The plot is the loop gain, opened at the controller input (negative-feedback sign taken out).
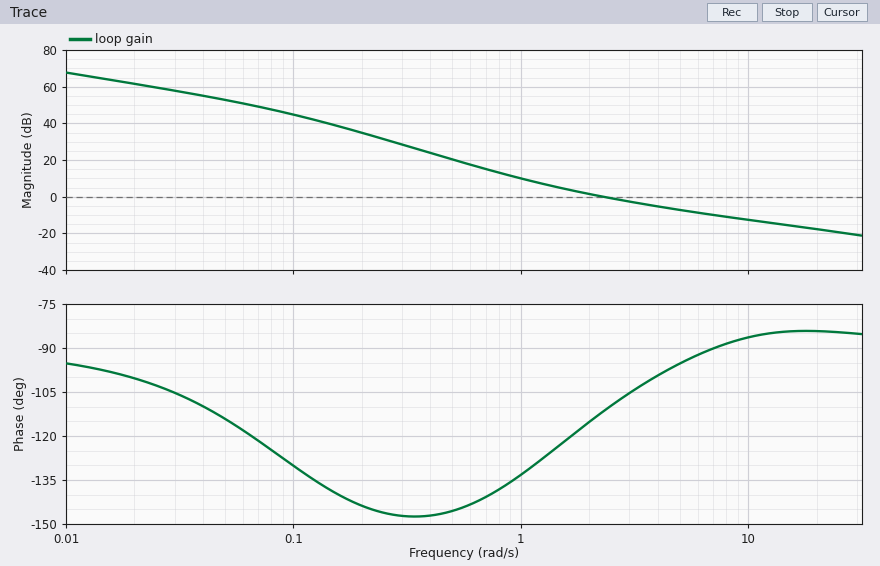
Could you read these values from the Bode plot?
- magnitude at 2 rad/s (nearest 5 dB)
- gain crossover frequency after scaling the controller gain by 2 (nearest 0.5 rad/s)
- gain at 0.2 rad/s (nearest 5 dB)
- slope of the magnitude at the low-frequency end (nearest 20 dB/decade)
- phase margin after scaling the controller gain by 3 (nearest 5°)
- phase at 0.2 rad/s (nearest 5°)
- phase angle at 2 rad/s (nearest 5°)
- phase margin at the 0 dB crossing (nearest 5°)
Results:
0 dB
4.5 rad/s
35 dB
-20 dB/decade
90°
-145°
-115°
70°
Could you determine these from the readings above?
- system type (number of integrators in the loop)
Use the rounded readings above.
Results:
1
